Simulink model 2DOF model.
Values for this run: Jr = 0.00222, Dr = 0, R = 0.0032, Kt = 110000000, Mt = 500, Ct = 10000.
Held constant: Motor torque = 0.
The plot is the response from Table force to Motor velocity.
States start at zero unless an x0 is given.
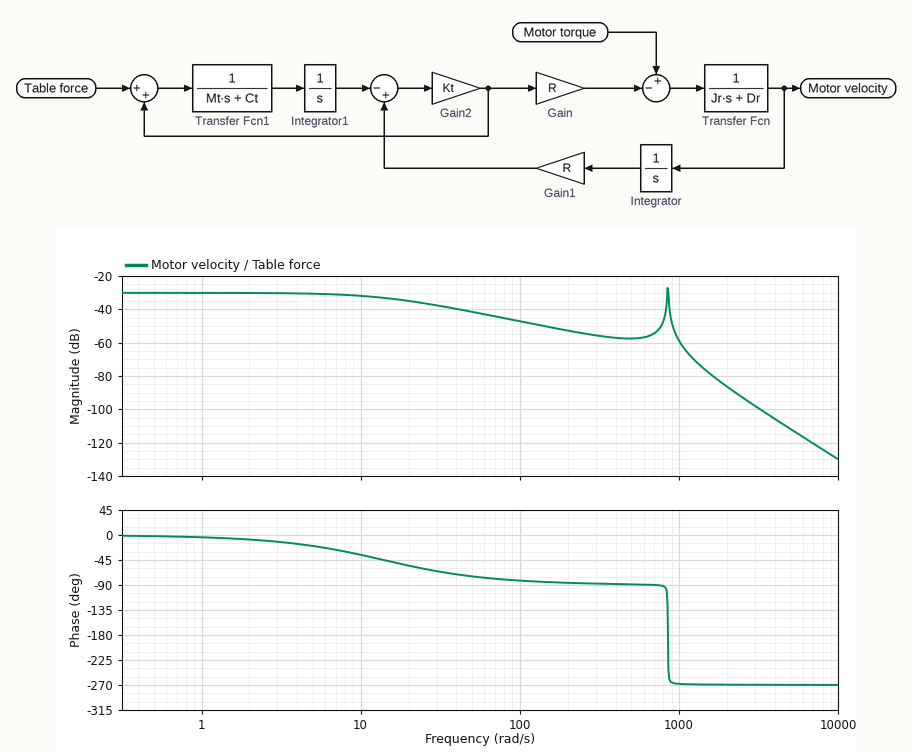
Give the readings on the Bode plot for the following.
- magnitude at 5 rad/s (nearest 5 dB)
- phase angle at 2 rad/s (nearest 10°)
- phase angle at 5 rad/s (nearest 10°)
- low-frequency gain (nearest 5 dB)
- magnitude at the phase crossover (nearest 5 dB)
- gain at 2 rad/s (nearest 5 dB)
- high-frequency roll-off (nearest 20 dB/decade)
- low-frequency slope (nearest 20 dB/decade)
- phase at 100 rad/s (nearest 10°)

-30 dB
-10°
-20°
-30 dB
-30 dB
-30 dB
-60 dB/decade
0 dB/decade
-80°
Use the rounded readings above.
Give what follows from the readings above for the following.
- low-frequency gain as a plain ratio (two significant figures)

0.032
